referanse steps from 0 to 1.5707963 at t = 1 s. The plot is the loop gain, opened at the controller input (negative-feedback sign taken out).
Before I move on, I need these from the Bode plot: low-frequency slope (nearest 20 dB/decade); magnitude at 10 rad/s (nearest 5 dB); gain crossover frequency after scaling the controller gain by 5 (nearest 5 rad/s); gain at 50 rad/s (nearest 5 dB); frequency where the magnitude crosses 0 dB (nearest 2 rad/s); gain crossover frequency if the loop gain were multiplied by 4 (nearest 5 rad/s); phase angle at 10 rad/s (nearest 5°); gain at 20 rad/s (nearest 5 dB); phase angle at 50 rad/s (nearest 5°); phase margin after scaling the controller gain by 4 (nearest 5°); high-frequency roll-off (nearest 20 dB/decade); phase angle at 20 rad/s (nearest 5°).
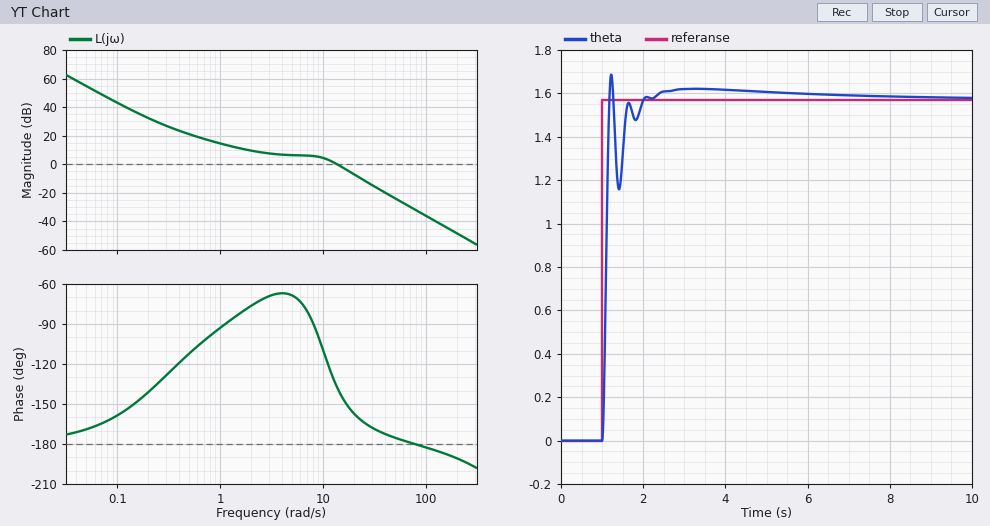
-40 dB/decade
5 dB
30 rad/s
-25 dB
14 rad/s
25 rad/s
-110°
-5 dB
-175°
15°
-40 dB/decade
-155°
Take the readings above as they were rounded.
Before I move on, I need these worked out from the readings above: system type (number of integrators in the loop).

2
